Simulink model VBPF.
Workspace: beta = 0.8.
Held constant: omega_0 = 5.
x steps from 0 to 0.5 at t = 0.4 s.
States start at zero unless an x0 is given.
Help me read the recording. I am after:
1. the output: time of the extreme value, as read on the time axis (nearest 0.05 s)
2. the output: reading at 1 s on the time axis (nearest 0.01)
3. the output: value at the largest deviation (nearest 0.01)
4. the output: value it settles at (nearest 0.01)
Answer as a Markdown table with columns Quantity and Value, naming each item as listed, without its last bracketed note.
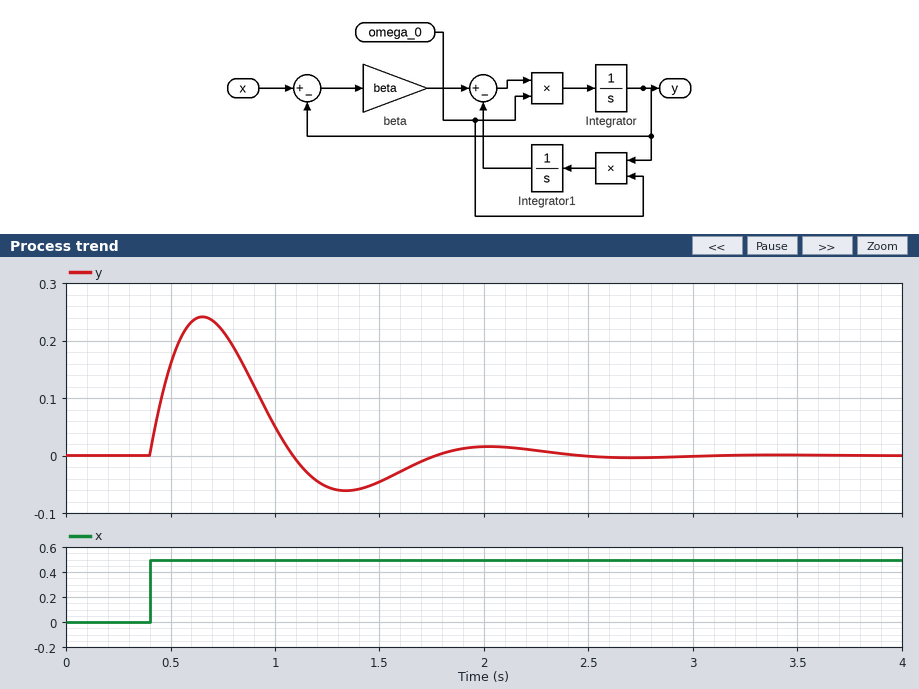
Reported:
| Quantity | Value |
|---|---|
| the output: time of the extreme value, as read on the time axis | 0.65 s |
| the output: reading at 1 s on the time axis | 0.05 |
| the output: value at the largest deviation | 0.24 |
| the output: value it settles at | 0.00 |
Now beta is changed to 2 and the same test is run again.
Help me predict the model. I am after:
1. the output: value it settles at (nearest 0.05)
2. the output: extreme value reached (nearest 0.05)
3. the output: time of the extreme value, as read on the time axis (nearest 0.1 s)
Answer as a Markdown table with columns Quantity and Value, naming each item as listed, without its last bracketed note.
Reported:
| Quantity | Value |
|---|---|
| the output: value it settles at | 0.00 |
| the output: extreme value reached | 0.35 |
| the output: time of the extreme value, as read on the time axis | 0.6 s |
